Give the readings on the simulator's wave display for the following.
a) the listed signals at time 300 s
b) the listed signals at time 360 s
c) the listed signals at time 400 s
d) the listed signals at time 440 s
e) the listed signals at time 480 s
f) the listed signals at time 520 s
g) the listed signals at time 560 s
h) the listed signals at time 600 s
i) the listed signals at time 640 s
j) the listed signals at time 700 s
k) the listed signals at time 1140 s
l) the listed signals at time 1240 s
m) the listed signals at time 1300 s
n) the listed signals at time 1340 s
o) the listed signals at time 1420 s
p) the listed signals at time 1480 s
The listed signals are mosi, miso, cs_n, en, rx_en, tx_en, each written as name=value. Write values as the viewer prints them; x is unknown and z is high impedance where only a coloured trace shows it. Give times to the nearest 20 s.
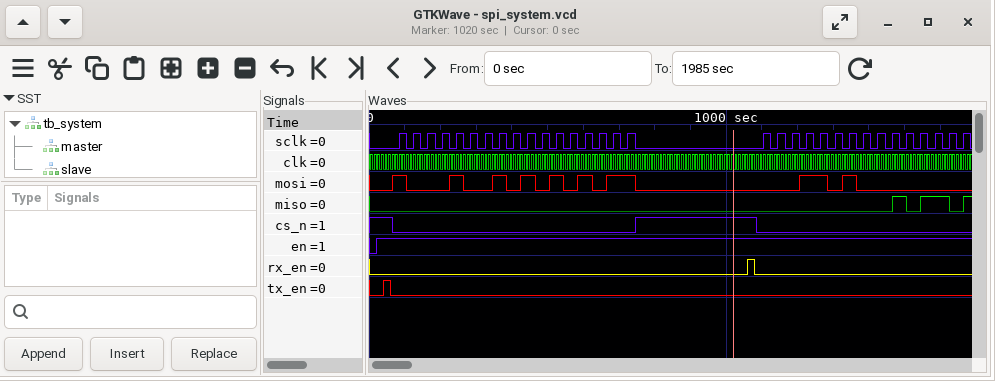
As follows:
mosi=0, miso=0, cs_n=0, en=1, rx_en=0, tx_en=0
mosi=1, miso=0, cs_n=0, en=1, rx_en=0, tx_en=0
mosi=0, miso=0, cs_n=0, en=1, rx_en=0, tx_en=0
mosi=1, miso=0, cs_n=0, en=1, rx_en=0, tx_en=0
mosi=0, miso=0, cs_n=0, en=1, rx_en=0, tx_en=0
mosi=1, miso=0, cs_n=0, en=1, rx_en=0, tx_en=0
mosi=0, miso=0, cs_n=0, en=1, rx_en=0, tx_en=0
mosi=1, miso=0, cs_n=0, en=1, rx_en=0, tx_en=0
mosi=0, miso=0, cs_n=0, en=1, rx_en=0, tx_en=0
mosi=1, miso=0, cs_n=0, en=1, rx_en=0, tx_en=0
mosi=0, miso=0, cs_n=0, en=1, rx_en=0, tx_en=0
mosi=1, miso=0, cs_n=0, en=1, rx_en=0, tx_en=0
mosi=0, miso=0, cs_n=0, en=1, rx_en=0, tx_en=0
mosi=1, miso=0, cs_n=0, en=1, rx_en=0, tx_en=0
mosi=0, miso=0, cs_n=0, en=1, rx_en=0, tx_en=0
mosi=0, miso=1, cs_n=0, en=1, rx_en=0, tx_en=0
